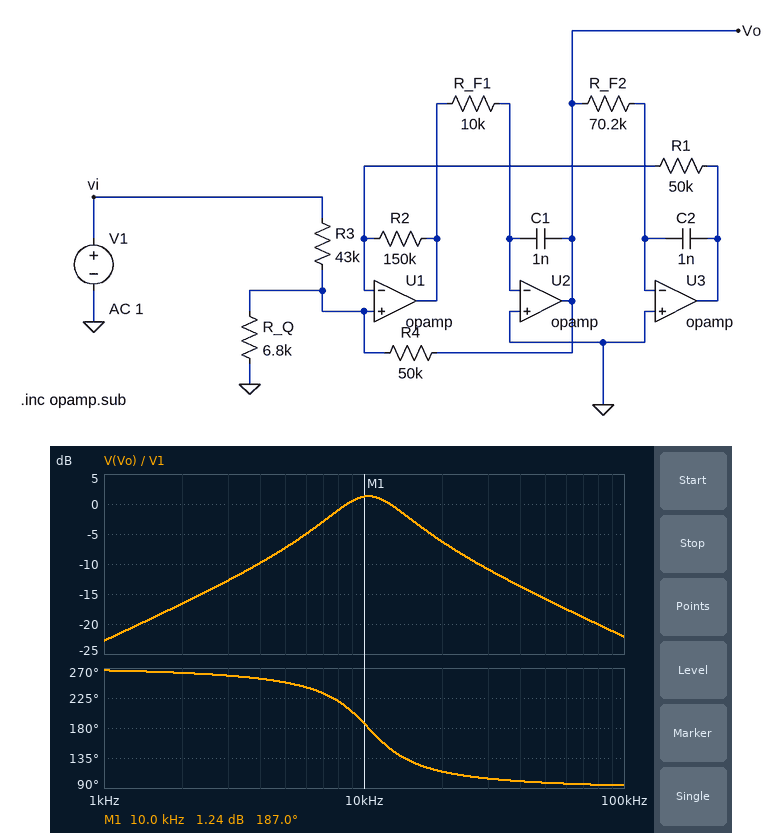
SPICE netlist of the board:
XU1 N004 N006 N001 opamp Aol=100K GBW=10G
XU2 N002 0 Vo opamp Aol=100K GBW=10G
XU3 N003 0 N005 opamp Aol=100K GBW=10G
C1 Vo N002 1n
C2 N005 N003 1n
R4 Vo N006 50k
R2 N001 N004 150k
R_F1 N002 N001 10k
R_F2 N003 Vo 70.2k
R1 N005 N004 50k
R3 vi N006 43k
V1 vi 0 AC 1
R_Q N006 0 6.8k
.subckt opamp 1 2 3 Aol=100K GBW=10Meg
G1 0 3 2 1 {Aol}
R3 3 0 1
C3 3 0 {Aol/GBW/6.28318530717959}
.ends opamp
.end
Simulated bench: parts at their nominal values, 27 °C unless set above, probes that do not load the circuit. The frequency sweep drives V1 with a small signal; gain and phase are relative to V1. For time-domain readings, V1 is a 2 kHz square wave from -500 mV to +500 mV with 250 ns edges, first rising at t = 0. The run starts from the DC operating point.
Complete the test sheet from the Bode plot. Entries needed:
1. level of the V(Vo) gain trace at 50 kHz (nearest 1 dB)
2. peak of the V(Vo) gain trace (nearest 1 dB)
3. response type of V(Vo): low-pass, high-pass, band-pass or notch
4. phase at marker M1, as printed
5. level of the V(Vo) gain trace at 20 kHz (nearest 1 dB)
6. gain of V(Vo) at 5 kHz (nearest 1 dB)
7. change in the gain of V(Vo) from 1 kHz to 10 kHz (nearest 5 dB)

-16 dB
1 dB
band-pass
187.0 deg
-6 dB
-7 dB
25 dB
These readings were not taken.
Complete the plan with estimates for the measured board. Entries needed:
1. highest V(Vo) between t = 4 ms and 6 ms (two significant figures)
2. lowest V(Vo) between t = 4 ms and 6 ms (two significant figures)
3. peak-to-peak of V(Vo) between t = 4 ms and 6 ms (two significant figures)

490 mV
-490 mV
990 mV
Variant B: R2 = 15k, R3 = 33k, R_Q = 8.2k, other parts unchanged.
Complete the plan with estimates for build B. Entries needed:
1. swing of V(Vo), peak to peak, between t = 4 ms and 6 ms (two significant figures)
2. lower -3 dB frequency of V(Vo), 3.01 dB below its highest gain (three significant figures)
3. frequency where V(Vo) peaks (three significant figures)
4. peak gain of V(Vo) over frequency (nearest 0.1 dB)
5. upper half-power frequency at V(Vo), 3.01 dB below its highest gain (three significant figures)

1.4 V
2.30 kHz
3.29 kHz
3.6 dB
4.70 kHz
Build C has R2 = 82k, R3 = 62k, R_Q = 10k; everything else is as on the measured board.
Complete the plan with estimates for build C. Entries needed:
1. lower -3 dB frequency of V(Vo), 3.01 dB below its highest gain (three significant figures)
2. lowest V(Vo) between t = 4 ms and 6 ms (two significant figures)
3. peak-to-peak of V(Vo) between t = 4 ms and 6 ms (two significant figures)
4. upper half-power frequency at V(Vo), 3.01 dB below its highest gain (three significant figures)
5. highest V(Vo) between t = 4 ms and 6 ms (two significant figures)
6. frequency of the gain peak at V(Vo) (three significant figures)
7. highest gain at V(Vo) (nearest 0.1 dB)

5.20 kHz
-390 mV
780 mV
11.4 kHz
390 mV
7.69 kHz
-1.9 dB
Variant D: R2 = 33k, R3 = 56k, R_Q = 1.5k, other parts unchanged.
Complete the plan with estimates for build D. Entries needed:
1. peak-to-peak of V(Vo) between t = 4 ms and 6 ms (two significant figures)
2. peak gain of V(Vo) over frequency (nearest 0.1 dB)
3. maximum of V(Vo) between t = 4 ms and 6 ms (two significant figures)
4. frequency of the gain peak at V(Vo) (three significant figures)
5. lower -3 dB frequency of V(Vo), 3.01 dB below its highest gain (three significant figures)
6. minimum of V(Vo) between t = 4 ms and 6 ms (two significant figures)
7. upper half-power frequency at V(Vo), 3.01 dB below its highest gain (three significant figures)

190 mV
-1.0 dB
95 mV
4.88 kHz
4.52 kHz
-95 mV
5.27 kHz
